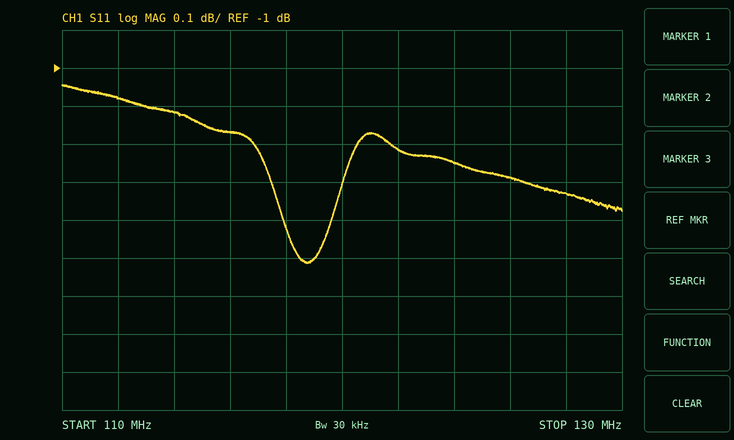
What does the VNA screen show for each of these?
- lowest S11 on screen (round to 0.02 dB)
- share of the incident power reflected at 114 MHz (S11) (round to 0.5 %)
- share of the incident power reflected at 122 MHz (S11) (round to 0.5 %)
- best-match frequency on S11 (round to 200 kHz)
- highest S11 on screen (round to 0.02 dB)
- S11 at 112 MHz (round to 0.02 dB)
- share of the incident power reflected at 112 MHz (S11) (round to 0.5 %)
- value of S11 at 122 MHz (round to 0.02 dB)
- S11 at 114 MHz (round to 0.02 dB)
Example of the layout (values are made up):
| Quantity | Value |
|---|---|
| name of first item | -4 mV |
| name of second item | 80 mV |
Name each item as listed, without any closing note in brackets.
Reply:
| Quantity | Value |
|---|---|
| lowest S11 on screen | -1.52 dB |
| share of the incident power reflected at 114 MHz (S11) | 77.5 % |
| share of the incident power reflected at 122 MHz (S11) | 75.5 % |
| best-match frequency on S11 | 118.8 MHz |
| highest S11 on screen | -1.04 dB |
| S11 at 112 MHz | -1.08 dB |
| share of the incident power reflected at 112 MHz (S11) | 78.0 % |
| value of S11 at 122 MHz | -1.22 dB |
| S11 at 114 MHz | -1.12 dB |
